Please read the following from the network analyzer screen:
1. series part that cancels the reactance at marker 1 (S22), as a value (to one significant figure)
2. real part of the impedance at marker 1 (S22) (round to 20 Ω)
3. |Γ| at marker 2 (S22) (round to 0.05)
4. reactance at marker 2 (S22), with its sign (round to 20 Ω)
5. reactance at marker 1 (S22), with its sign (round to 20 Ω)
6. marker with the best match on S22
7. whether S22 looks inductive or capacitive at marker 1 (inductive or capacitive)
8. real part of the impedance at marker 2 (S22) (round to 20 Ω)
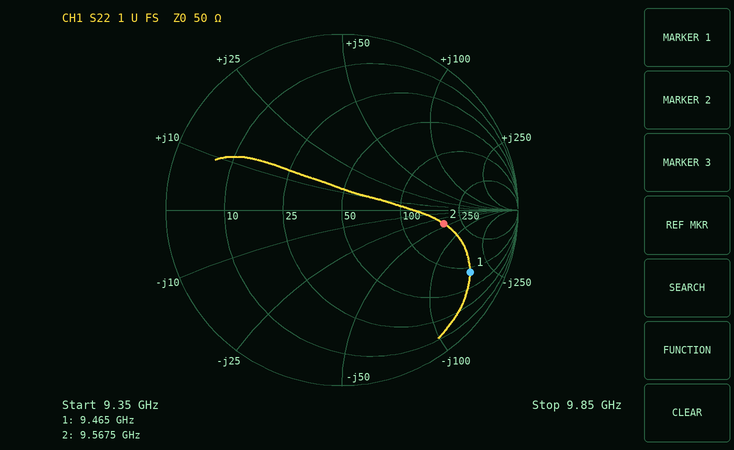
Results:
3 nH
80 Ω
0.60
-40 Ω
-180 Ω
marker 2
capacitive
180 Ω
